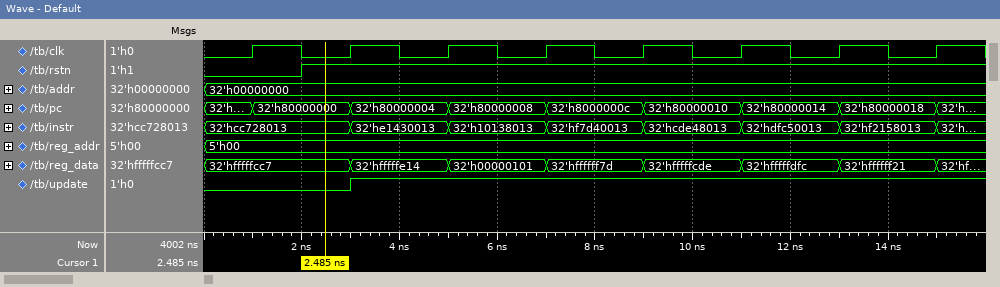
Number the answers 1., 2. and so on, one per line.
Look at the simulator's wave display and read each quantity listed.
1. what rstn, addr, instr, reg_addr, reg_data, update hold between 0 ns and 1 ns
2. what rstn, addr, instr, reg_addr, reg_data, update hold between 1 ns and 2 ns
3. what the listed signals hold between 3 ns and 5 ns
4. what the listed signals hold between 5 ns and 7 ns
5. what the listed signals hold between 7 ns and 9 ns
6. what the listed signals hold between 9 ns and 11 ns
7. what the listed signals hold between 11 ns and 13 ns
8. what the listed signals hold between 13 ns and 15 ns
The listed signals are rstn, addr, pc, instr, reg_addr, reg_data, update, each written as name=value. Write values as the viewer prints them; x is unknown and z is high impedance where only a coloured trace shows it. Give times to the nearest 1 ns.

1. rstn=0, addr=32'h00000000, instr=32'hcc728013, reg_addr=5'h00, reg_data=32'hfffffcc7, update=0
2. rstn=0, addr=32'h00000000, instr=32'hcc728013, reg_addr=5'h00, reg_data=32'hfffffcc7, update=0
3. rstn=1, addr=32'h00000000, pc=32'h80000004, instr=32'he1430013, reg_addr=5'h00, reg_data=32'hfffffe14, update=1
4. rstn=1, addr=32'h00000000, pc=32'h80000008, instr=32'h10138013, reg_addr=5'h00, reg_data=32'h00000101, update=1
5. rstn=1, addr=32'h00000000, pc=32'h8000000c, instr=32'hf7d40013, reg_addr=5'h00, reg_data=32'hffffff7d, update=1
6. rstn=1, addr=32'h00000000, pc=32'h80000010, instr=32'hcde48013, reg_addr=5'h00, reg_data=32'hfffffcde, update=1
7. rstn=1, addr=32'h00000000, pc=32'h80000014, instr=32'hdfc50013, reg_addr=5'h00, reg_data=32'hfffffdfc, update=1
8. rstn=1, addr=32'h00000000, pc=32'h80000018, instr=32'hf2158013, reg_addr=5'h00, reg_data=32'hffffff21, update=1
